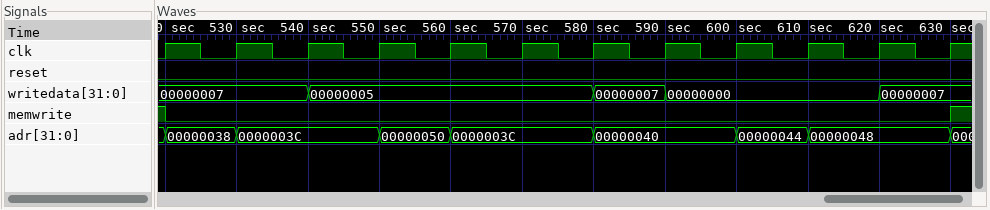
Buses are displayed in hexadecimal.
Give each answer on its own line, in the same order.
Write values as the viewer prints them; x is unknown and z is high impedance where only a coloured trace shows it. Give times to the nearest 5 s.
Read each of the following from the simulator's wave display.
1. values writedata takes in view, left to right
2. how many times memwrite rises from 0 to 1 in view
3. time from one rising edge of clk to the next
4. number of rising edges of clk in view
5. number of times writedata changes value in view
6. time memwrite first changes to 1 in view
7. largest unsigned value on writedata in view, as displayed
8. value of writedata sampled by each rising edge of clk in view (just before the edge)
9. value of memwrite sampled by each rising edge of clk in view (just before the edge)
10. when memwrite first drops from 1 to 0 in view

00000007, 00000005, 00000007, 00000000, 00000007
1
10 s
12
4
630 s
00000007
00000007, 00000007, 00000007, 00000005, 00000005, 00000005, 00000005, 00000007, 00000000, 00000000, 00000000, 00000007
1 0 0 0 0 0 0 0 0 0 0 0
520 s
